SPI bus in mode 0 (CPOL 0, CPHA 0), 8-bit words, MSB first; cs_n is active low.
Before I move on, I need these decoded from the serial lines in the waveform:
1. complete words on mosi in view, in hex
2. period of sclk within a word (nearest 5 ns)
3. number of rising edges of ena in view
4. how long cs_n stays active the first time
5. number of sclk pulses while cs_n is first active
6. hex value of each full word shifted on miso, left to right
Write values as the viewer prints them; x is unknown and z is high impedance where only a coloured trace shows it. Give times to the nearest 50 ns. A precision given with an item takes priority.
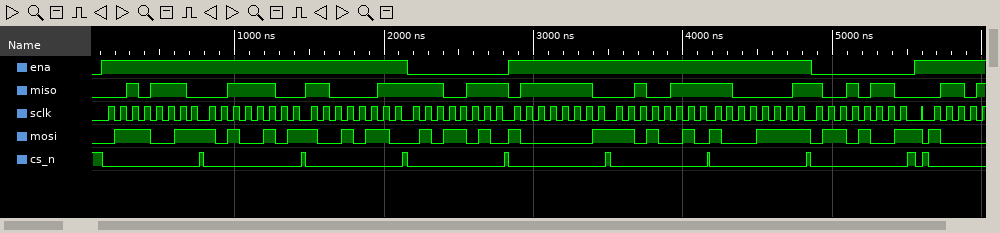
73, A5, 96, 5A, 81, D2, 8F, 69
80 ns
3
650 ns
8
2E, 3C, C3, E7, 7E, 27, C1, 96
